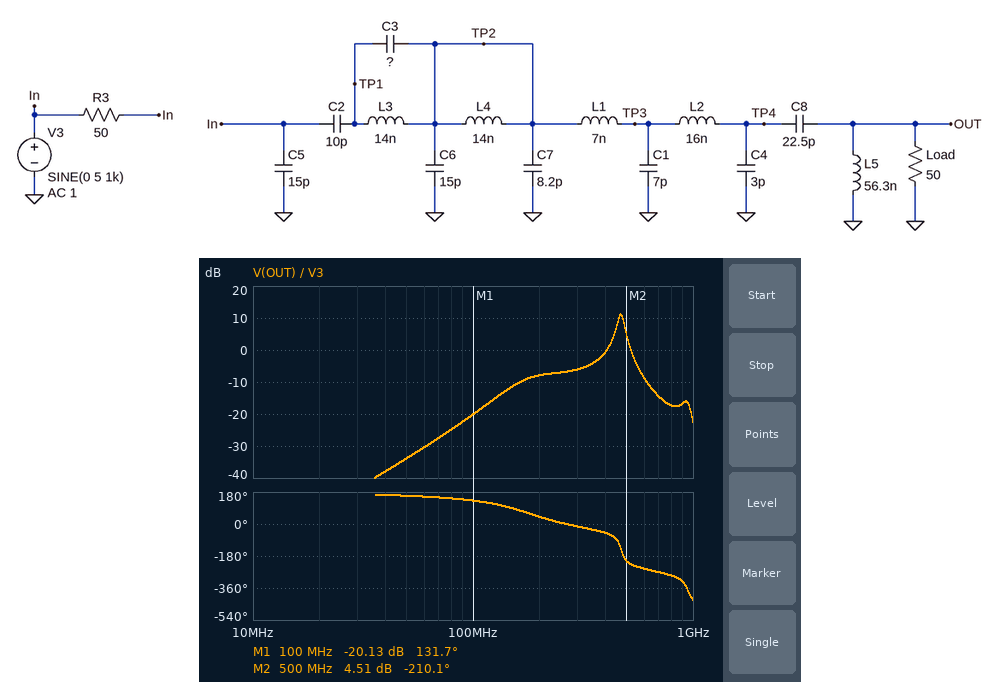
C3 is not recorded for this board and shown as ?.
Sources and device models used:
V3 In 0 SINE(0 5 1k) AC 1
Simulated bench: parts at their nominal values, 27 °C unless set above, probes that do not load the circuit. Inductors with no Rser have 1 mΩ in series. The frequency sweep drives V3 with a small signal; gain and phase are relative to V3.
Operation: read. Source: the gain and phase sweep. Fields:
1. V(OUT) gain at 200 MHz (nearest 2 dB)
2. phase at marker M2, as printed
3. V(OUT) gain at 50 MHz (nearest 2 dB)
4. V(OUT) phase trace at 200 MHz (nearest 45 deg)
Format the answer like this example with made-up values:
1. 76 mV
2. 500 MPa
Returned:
1. -8 dB
2. -210.1 deg
3. -34 dB
4. 45 deg
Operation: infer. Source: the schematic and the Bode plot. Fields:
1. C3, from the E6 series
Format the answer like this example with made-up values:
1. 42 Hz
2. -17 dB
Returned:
1. 1 pF
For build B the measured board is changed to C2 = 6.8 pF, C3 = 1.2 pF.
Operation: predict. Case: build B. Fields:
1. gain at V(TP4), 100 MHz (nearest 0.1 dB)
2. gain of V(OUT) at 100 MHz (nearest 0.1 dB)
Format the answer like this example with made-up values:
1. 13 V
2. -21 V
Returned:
1. -18.5 dB
2. -23.3 dB
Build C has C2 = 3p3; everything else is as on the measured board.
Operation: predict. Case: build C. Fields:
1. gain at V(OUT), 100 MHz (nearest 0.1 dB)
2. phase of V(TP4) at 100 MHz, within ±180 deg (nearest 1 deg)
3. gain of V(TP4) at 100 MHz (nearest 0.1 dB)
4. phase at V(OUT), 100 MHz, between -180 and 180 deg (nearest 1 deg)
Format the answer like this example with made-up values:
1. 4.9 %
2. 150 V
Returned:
1. -29.4 dB
2. 8 deg
3. -24.6 dB
4. 133 deg
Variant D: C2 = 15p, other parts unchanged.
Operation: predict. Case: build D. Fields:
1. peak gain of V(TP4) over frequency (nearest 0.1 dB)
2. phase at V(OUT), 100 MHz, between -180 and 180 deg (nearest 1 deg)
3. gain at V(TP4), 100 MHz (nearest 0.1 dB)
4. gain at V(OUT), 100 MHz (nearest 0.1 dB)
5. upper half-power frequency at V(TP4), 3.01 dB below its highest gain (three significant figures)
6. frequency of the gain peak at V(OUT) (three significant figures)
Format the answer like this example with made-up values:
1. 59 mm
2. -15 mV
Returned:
1. 9.7 dB
2. 131 deg
3. -12.1 dB
4. -16.9 dB
5. 439 MHz
6. 417 MHz
